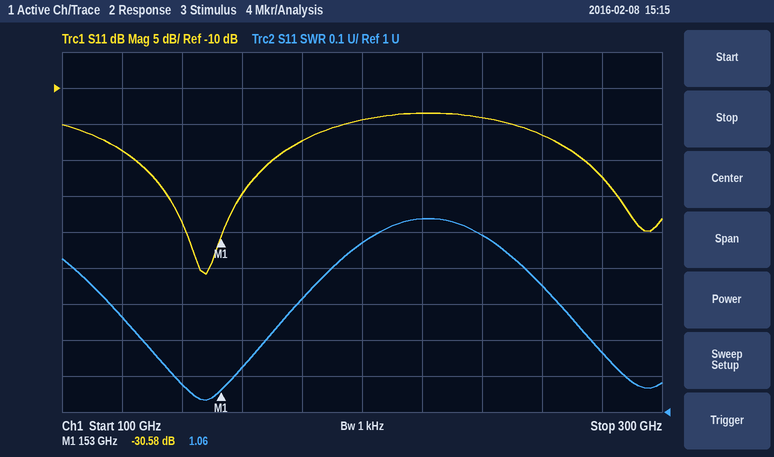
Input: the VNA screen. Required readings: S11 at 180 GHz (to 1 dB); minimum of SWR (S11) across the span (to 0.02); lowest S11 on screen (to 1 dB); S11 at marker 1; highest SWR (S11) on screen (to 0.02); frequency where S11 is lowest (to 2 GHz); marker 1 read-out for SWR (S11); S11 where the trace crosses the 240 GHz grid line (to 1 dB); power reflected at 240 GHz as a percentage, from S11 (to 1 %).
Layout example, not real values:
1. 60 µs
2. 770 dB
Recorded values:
1. -17 dB
2. 1.04
3. -36 dB
4. -30.58 dB
5. 1.54
6. 148 GHz
7. 1.06
8. -14 dB
9. 4 %
